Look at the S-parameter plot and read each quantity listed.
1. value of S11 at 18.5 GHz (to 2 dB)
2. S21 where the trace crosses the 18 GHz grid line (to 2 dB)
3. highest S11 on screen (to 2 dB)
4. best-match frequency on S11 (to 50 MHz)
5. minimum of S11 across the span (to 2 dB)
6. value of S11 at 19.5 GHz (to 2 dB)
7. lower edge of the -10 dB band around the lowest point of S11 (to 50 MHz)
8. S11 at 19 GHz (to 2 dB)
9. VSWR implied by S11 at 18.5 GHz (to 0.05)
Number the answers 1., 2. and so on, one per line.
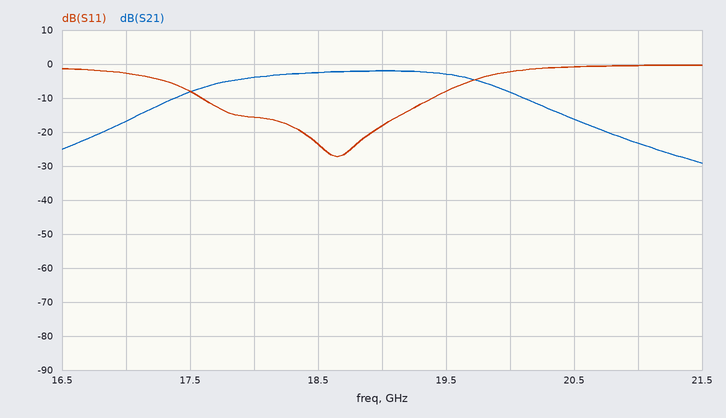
1. -24 dB
2. -4 dB
3. 0 dB
4. 18.65 GHz
5. -28 dB
6. -8 dB
7. 17.60 GHz
8. -18 dB
9. 1.15
